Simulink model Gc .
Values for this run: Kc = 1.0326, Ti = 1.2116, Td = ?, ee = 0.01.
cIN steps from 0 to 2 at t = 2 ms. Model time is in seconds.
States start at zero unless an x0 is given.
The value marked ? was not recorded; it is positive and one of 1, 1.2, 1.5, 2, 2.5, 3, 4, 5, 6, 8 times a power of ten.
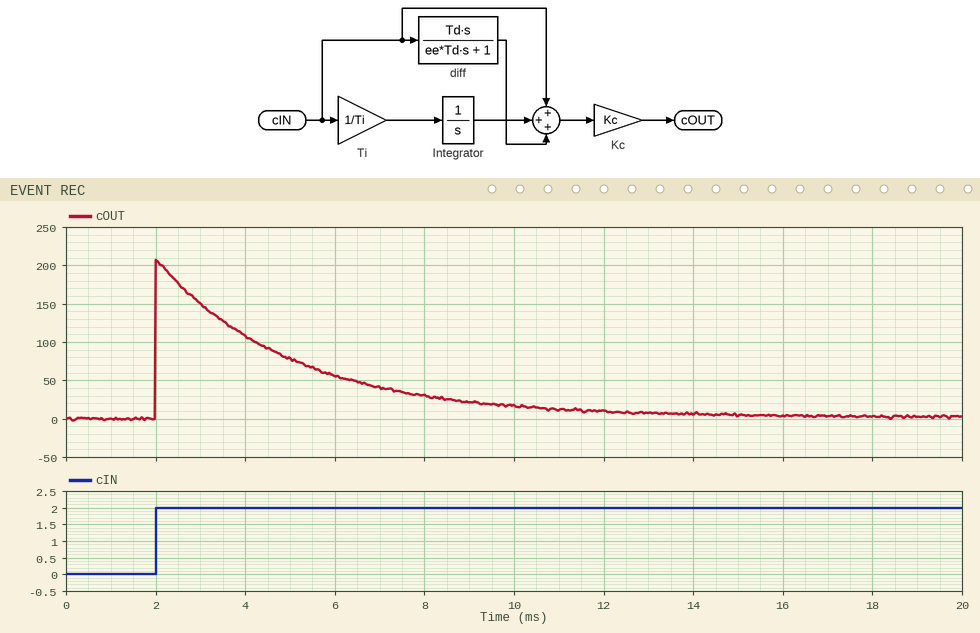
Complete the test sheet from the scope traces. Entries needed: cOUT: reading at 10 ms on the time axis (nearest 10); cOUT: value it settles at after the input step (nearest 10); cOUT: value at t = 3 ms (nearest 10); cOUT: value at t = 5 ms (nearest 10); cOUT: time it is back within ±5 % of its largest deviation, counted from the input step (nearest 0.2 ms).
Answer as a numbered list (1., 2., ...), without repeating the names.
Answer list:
1. 20
2. 0
3. 150
4. 80
5. 9.0 ms
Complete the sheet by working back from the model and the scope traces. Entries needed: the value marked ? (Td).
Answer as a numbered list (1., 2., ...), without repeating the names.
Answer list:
1. 0.3
